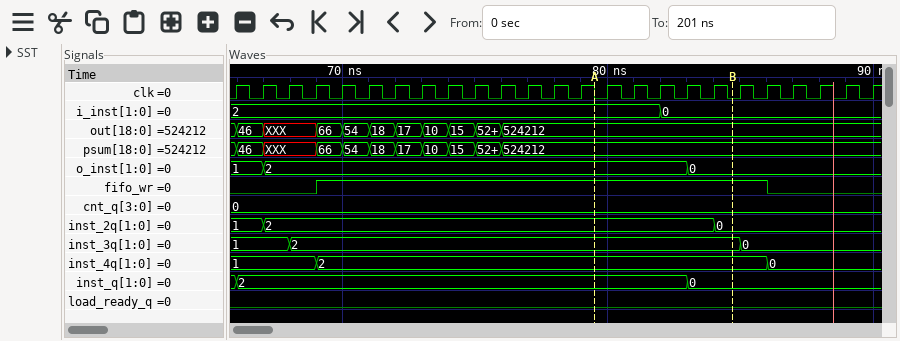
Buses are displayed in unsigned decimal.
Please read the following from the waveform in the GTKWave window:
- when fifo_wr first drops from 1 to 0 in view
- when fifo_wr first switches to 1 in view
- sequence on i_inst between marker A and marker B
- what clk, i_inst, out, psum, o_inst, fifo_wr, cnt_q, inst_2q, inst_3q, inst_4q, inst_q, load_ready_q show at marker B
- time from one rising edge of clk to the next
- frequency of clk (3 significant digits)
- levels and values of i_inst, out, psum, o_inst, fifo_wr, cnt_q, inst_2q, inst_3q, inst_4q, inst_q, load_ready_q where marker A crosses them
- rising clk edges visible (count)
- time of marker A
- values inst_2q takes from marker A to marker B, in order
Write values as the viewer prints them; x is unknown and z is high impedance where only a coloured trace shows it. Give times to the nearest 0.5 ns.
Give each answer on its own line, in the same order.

86 ns
69 ns
2, 0
clk=0, i_inst=0, out=524212, psum=524212, o_inst=0, fifo_wr=1, cnt_q=0, inst_2q=0, inst_3q=2, inst_4q=2, inst_q=0, load_ready_q=0
1 ns
1.00 GHz
i_inst=2, out=524212, psum=524212, o_inst=2, fifo_wr=1, cnt_q=0, inst_2q=2, inst_3q=2, inst_4q=2, inst_q=2, load_ready_q=0
25
79.5 ns
2, 0
